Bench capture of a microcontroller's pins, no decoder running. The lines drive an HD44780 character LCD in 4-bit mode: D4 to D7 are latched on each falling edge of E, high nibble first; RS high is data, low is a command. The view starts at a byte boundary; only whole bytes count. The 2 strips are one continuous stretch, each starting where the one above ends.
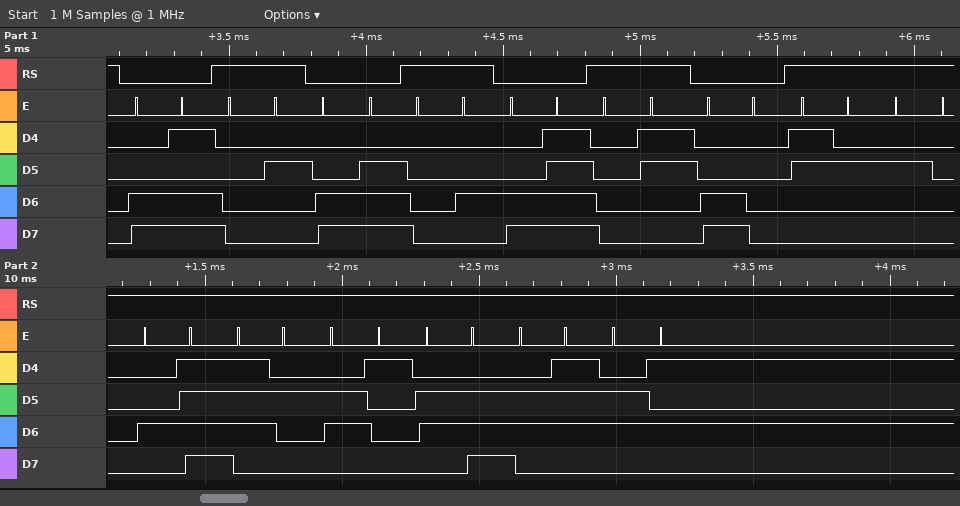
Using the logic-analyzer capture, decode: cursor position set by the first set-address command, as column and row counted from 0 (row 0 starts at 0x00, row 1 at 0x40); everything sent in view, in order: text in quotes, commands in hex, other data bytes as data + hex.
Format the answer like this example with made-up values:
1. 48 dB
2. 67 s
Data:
1. column 13, row 1
2. 0xCD data 02 0xCE data 04 0xCF data 03 0xC0 "2 Orange"
